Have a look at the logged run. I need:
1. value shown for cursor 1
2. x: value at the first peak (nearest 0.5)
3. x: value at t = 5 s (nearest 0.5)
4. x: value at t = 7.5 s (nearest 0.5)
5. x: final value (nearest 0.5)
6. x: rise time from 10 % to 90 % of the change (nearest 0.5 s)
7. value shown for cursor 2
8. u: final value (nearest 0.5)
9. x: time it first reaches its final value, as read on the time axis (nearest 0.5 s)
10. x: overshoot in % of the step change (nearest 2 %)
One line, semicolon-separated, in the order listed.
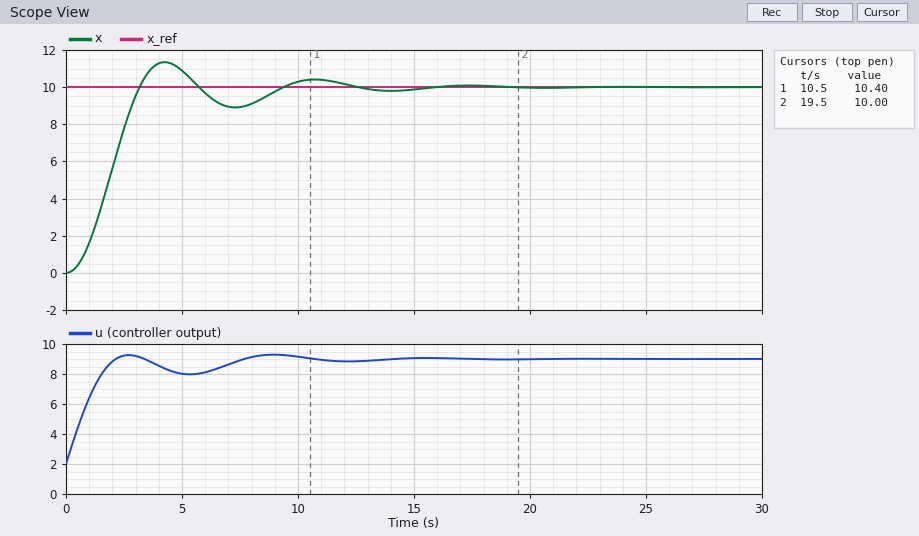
10.40; 11.5; 11.0; 9.0; 10.0; 2.0 s; 10.00; 9.0; 3.0 s; 14 %
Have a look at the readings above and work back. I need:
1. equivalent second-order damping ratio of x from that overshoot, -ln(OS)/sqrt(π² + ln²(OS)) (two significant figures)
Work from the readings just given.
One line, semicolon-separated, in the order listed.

0.53
